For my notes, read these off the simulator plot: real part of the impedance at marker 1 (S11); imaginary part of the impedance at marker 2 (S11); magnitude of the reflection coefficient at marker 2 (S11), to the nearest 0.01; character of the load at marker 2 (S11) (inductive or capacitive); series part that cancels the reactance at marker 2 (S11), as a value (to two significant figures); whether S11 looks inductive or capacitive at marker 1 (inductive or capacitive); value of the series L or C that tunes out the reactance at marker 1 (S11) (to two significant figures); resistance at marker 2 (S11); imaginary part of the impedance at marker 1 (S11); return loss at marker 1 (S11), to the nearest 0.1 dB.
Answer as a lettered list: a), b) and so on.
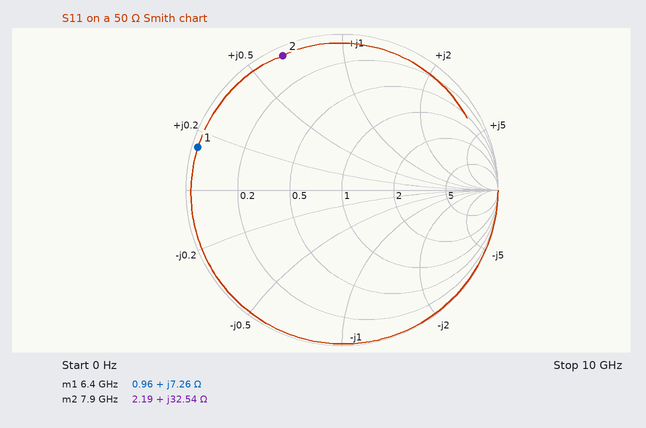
a) 0.96 Ω
b) +32.54 Ω
c) 0.94
d) inductive
e) 620 fF
f) inductive
g) 3.4 pF
h) 2.19 Ω
i) +7.26 Ω
j) 0.3 dB
